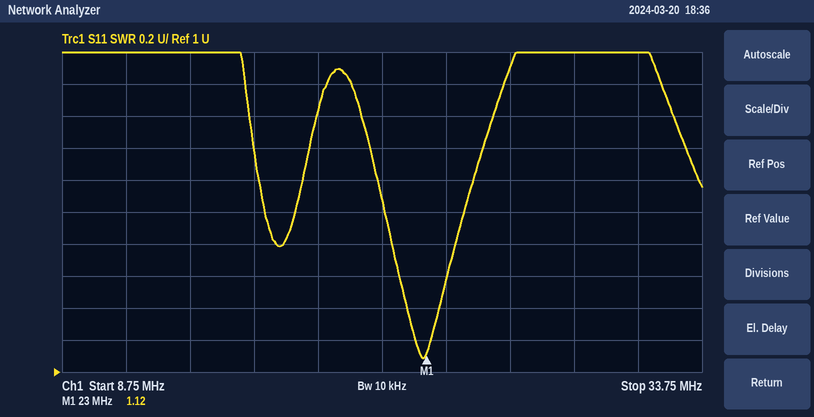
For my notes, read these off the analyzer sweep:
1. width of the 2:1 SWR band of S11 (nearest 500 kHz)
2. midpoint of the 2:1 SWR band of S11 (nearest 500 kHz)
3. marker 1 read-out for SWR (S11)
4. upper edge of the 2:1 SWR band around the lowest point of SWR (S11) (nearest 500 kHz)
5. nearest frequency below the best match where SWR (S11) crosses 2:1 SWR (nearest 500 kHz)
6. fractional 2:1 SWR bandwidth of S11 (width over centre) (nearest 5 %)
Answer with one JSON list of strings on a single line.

["3.0 MHz", "23.0 MHz", "1.12", "24.5 MHz", "21.5 MHz", "15 %"]
